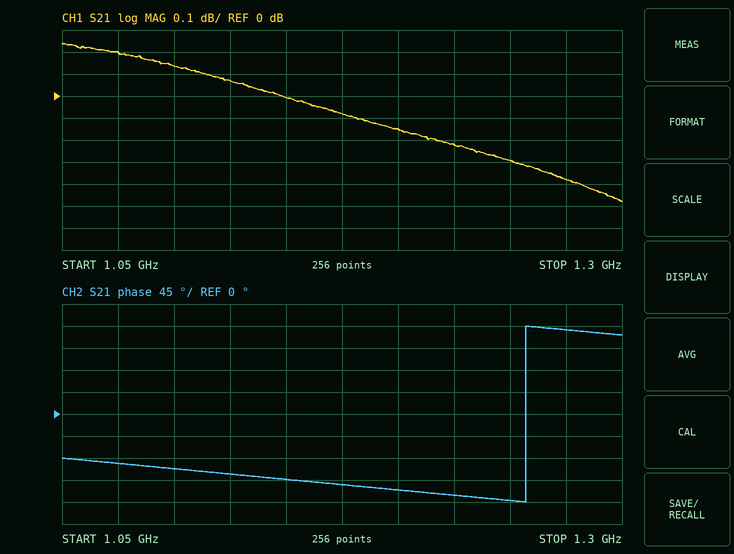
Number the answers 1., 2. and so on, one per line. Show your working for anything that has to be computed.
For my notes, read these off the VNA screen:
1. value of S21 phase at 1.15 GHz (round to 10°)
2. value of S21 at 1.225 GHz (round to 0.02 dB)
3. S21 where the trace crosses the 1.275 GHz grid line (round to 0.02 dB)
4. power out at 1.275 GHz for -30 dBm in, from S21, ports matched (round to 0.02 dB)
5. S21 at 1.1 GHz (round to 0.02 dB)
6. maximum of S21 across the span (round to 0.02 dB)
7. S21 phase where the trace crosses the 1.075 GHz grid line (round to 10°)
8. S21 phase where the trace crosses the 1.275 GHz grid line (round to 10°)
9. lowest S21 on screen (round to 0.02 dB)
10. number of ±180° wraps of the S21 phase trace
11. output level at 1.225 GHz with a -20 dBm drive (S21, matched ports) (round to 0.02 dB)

1. -130°
2. -0.22 dB
3. -0.38 dB
4. -30 dBm + (-0.38 dB) = -30.38 dBm
5. 0.14 dB
6. 0.24 dB
7. -100°
8. 170°
9. -0.48 dB
10. 1
11. -20 dBm + (-0.22 dB) = -20.22 dBm
